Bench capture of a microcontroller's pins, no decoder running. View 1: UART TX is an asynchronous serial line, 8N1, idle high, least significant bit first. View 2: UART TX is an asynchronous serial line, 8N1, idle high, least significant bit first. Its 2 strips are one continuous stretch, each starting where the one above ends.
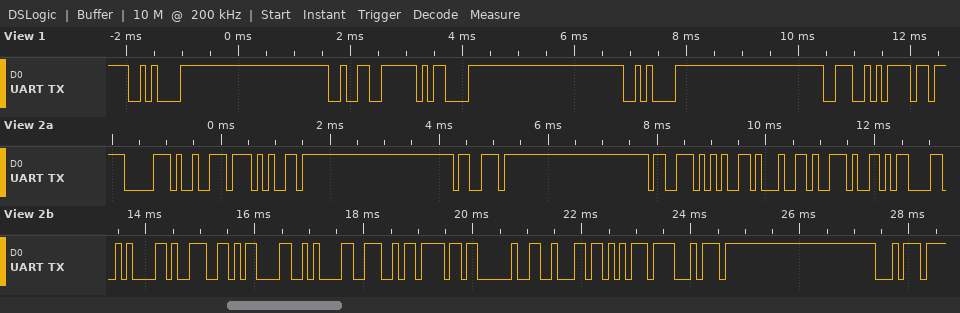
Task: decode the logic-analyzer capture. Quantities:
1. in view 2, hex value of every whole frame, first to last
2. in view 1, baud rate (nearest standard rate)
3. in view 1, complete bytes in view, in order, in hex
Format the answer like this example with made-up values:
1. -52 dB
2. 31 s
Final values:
1. 70 72 65 73 73 65 64 2E 0D 0A 39 0D 0A 4E 6F 20 62 75 74 74
2. 9600 baud
3. 0x0A 0x32 0x0D 0x0A 0x4E 0x6F
